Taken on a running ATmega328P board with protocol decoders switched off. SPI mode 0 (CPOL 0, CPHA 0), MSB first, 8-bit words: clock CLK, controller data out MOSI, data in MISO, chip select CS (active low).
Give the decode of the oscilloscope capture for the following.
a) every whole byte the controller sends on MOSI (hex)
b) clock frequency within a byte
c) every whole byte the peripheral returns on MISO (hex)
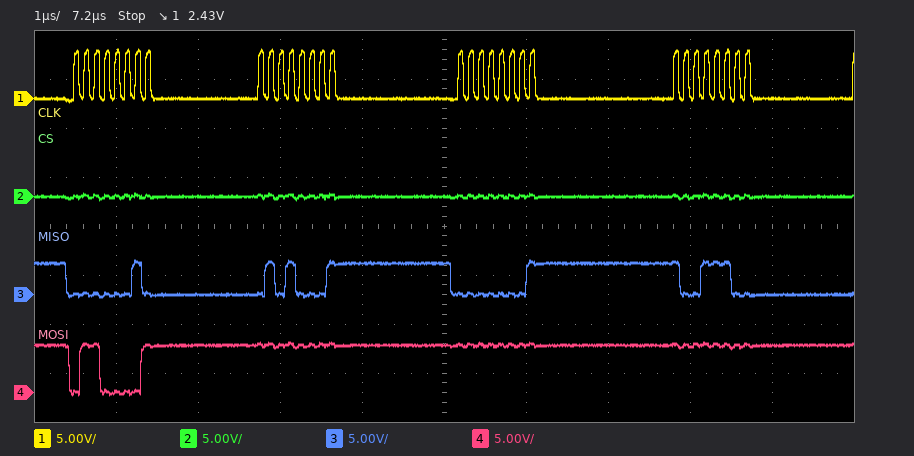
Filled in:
0x61 0xFF 0xFF 0xFF
8 MHz
0x02 0x51 0x01 0x9C
